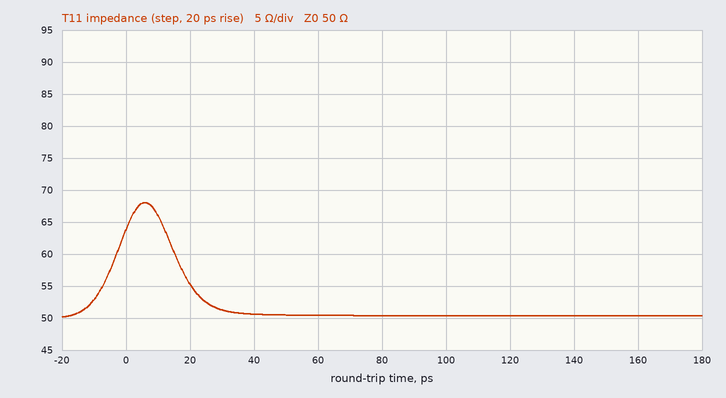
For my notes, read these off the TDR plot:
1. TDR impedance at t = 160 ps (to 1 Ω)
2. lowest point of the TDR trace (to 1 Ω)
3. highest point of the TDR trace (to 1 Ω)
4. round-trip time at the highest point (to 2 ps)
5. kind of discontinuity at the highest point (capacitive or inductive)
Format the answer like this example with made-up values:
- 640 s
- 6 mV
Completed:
- 50 Ω
- 50 Ω
- 68 Ω
- 6 ps
- inductive
